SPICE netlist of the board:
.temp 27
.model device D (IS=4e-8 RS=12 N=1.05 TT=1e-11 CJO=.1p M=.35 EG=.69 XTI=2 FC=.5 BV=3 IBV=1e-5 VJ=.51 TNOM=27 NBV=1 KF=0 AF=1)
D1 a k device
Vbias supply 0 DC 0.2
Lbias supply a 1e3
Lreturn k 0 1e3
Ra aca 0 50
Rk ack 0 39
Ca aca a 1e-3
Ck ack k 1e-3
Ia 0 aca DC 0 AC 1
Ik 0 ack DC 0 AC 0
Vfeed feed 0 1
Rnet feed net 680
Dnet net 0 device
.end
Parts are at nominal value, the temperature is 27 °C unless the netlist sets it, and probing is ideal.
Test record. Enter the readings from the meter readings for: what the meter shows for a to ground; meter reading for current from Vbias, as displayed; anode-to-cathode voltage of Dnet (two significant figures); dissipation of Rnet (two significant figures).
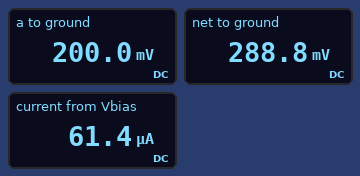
200.0 mV
61.4 µA
290 mV
740 µW
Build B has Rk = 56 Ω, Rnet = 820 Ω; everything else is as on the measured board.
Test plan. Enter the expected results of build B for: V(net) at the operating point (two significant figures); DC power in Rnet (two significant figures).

280 mV
630 µW
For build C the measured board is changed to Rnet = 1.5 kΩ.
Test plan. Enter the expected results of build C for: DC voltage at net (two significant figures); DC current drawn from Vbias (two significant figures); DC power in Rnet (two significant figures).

260 mV
61 µA
360 µW
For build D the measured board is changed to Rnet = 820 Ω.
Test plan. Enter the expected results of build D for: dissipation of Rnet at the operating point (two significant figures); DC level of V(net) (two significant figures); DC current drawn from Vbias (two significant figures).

630 µW
280 mV
61 µA
